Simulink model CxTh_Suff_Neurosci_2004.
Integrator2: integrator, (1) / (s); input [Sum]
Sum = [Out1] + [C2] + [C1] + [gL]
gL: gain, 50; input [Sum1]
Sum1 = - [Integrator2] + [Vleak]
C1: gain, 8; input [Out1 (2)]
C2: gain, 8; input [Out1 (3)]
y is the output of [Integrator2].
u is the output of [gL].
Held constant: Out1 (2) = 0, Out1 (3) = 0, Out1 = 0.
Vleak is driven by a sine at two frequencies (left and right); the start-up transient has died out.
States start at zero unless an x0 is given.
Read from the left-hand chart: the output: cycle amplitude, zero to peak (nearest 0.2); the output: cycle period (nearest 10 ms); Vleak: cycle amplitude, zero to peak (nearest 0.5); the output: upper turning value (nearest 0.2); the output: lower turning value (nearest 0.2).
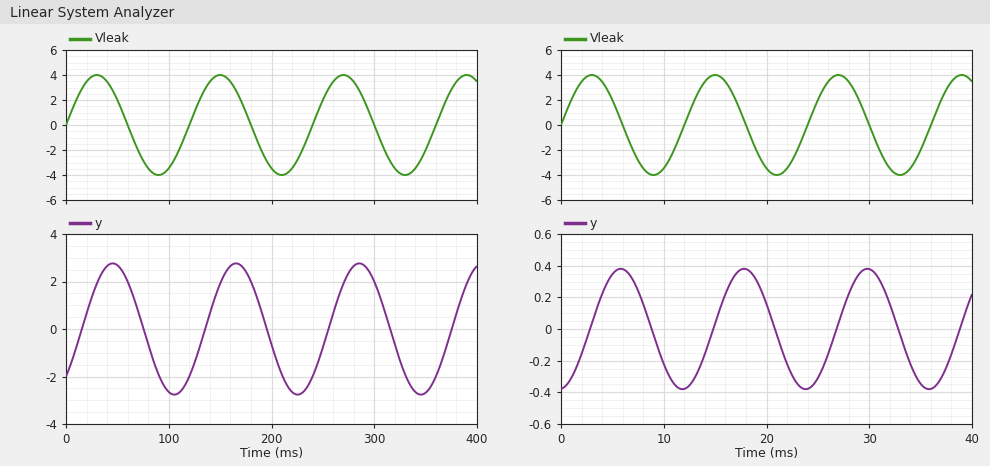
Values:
2.8
120 ms
4.0
2.8
-2.8
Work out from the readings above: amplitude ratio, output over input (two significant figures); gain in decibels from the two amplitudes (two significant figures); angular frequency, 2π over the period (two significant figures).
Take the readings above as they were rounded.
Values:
0.70
-3.1 dB
0.052 rad/ms
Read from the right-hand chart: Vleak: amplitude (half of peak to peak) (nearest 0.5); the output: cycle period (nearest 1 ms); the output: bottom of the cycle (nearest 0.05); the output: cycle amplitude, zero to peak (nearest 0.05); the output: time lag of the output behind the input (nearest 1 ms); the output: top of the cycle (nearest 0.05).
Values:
4.0
12 ms
-0.40
0.40
3 ms
0.40
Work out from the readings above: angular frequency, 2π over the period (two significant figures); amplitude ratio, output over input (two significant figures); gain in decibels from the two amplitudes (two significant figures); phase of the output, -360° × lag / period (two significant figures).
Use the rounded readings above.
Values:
0.52 rad/ms
0.10
-20 dB
-90°
